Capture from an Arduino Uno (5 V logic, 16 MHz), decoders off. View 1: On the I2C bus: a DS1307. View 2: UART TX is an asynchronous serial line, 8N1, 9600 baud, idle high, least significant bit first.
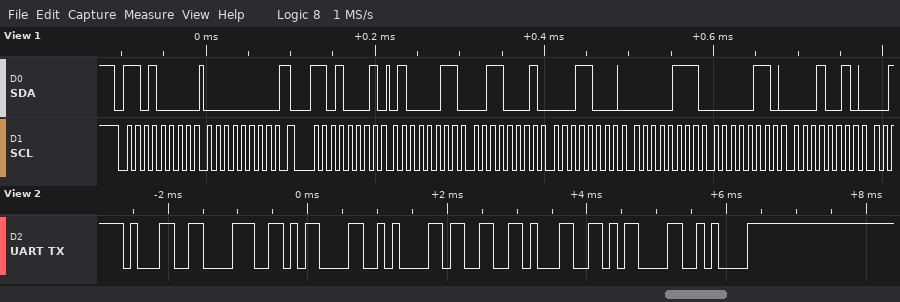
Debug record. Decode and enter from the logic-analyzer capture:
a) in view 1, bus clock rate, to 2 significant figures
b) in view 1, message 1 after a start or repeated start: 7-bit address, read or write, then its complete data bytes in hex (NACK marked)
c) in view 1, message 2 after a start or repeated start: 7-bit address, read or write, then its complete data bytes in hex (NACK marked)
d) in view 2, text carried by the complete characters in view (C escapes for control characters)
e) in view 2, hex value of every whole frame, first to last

100 kHz
0x68 write: 00
0x68 read: 43 31 18 07 06 12
"18\r\n31\r\n"
0x31 0x38 0x0D 0x0A 0x33 0x31 0x0D 0x0A
